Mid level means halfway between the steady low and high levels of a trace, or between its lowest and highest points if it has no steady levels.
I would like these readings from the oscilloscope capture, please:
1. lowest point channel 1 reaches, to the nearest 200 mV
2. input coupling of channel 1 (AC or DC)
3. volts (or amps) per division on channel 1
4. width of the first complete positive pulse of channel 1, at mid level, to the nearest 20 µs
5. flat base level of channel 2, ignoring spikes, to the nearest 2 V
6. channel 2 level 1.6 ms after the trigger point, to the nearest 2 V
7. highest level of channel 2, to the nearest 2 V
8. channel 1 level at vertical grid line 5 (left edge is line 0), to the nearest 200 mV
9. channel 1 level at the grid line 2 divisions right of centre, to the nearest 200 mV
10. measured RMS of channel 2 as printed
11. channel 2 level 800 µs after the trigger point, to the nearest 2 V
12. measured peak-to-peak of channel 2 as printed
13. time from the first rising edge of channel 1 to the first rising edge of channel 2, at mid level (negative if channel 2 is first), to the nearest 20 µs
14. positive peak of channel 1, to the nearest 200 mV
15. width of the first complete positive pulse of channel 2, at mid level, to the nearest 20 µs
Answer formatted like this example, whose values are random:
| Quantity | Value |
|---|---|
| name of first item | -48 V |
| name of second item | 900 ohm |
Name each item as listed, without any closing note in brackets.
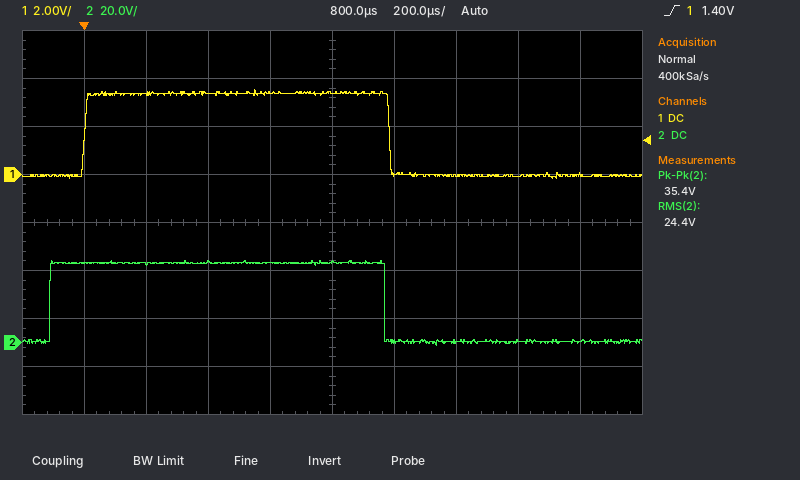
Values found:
| Quantity | Value |
|---|---|
| lowest point channel 1 reaches, to the nearest 200 mV | -200 mV |
| input coupling of channel 1 | DC |
| volts (or amps) per division on channel 1 | 2 V |
| width of the first complete positive pulse of channel 1, at mid level, to the nearest 20 µs | 980 µs |
| flat base level of channel 2, ignoring spikes, to the nearest 2 V | 0 V |
| channel 2 level 1.6 ms after the trigger point, to the nearest 2 V | 0 V |
| highest level of channel 2, to the nearest 2 V | 34 V |
| channel 1 level at vertical grid line 5 (left edge is line 0), to the nearest 200 mV | 3.4 V |
| channel 1 level at the grid line 2 divisions right of centre, to the nearest 200 mV | 0.0 V |
| measured RMS of channel 2 as printed | 24.4 V |
| channel 2 level 800 µs after the trigger point, to the nearest 2 V | 34 V |
| measured peak-to-peak of channel 2 as printed | 35.4 V |
| time from the first rising edge of channel 1 to the first rising edge of channel 2, at mid level (negative if channel 2 is first), to the nearest 20 µs | -120 µs |
| positive peak of channel 1, to the nearest 200 mV | 3.6 V |
| width of the first complete positive pulse of channel 2, at mid level, to the nearest 20 µs | 1.08 ms |
